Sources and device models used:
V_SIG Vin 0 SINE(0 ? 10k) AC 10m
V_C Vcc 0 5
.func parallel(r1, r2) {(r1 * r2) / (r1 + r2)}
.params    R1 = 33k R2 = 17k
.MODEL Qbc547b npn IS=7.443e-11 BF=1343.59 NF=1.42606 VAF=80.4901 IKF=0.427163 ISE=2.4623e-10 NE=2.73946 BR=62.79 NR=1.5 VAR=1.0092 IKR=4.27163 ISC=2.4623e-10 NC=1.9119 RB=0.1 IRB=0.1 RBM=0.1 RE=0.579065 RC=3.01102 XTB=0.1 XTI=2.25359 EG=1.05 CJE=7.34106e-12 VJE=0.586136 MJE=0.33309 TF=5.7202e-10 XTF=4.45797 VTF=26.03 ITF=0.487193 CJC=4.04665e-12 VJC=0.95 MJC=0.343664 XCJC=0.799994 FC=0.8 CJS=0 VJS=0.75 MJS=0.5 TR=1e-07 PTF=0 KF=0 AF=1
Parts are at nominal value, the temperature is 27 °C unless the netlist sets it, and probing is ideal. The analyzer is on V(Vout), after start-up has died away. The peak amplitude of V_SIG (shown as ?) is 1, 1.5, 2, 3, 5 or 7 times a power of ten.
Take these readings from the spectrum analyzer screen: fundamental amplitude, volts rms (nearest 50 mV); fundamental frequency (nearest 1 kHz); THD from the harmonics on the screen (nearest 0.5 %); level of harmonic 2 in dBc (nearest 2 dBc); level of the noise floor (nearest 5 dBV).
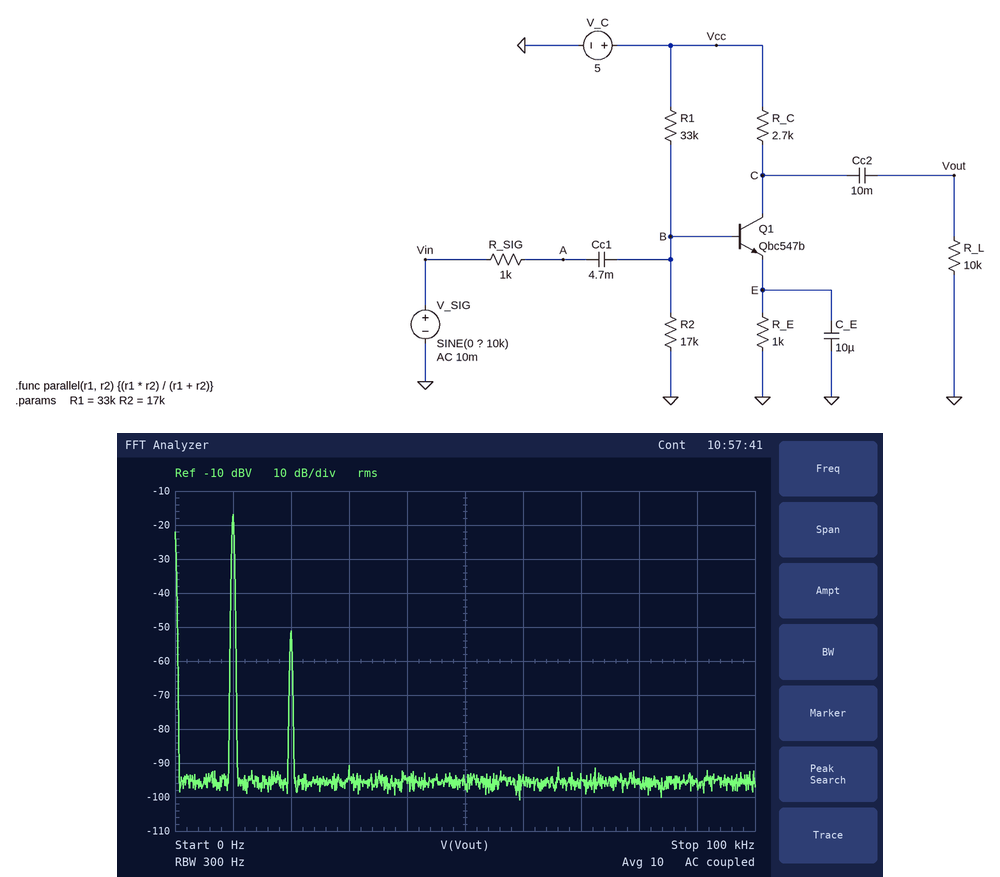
150 mV
10 kHz
2.0 %
-34 dBc
-95 dBV
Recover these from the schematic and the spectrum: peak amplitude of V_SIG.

5 mV
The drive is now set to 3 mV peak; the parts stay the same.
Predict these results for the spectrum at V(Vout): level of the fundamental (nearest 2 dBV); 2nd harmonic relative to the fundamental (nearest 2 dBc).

-22 dBV
-38 dBc
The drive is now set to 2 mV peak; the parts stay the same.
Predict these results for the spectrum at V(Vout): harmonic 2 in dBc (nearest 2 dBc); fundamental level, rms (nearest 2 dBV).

-42 dBc
-24 dBV
